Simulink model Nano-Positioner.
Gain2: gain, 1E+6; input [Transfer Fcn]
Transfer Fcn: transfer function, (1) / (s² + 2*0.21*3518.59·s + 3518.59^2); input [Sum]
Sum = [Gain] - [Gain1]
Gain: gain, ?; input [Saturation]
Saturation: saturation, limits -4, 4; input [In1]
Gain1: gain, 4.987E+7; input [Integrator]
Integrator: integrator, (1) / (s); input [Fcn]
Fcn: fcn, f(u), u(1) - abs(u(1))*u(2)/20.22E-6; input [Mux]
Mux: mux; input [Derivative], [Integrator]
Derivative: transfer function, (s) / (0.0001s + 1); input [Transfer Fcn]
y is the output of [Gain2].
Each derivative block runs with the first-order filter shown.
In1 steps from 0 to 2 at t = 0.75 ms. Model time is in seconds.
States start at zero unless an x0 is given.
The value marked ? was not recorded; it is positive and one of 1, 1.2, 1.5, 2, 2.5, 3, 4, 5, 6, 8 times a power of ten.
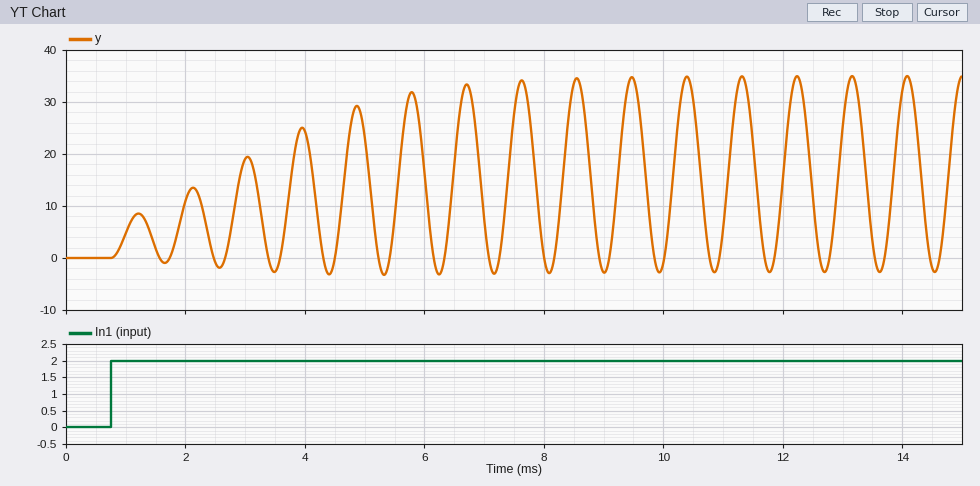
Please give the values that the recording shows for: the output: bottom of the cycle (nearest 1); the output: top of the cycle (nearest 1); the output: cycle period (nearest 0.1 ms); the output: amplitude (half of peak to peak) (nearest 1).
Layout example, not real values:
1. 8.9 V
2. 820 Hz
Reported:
1. -3
2. 35
3. 0.9 ms
4. 19
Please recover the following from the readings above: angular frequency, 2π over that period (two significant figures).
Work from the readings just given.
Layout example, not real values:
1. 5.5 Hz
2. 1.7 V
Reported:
1. 7.0 rad/ms
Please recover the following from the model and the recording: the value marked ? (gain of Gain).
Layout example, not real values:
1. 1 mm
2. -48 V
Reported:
1. 100
